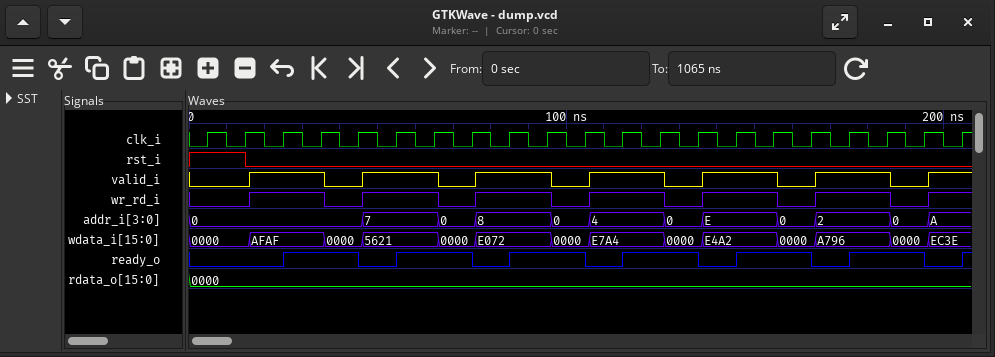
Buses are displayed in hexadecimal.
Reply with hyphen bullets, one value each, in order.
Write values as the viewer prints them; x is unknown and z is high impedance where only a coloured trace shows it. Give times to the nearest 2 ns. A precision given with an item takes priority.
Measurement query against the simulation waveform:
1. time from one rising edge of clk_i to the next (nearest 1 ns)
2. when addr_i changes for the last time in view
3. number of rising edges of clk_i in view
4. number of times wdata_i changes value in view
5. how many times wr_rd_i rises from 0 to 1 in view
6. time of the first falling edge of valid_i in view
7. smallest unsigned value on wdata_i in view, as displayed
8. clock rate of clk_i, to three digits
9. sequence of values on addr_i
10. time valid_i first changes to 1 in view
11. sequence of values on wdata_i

- 10 ns
- 196 ns
- 21
- 13
- 7
- 36 ns
- 0000
- 100 MHz
- 0, 7, 0, 8, 0, 4, 0, E, 0, 2, 0, A
- 16 ns
- 0000, AFAF, 0000, 5621, 0000, E072, 0000, E7A4, 0000, E4A2, 0000, A796, 0000, EC3E
